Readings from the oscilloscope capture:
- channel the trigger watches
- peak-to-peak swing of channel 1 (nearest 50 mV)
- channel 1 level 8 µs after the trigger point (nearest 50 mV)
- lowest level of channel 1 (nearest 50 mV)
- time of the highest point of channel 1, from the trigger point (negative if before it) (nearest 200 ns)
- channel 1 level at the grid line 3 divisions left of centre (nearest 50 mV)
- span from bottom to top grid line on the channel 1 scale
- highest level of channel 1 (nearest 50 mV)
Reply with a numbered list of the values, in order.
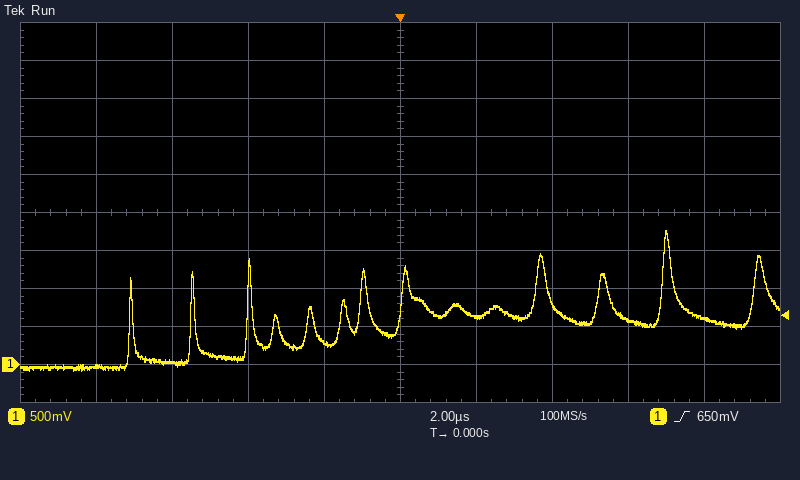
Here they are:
1. channel 1
2. 1.85 V
3. 600 mV
4. -100 mV
5. +7.0 µs
6. 50 mV
7. 5 V
8. 1.75 V
